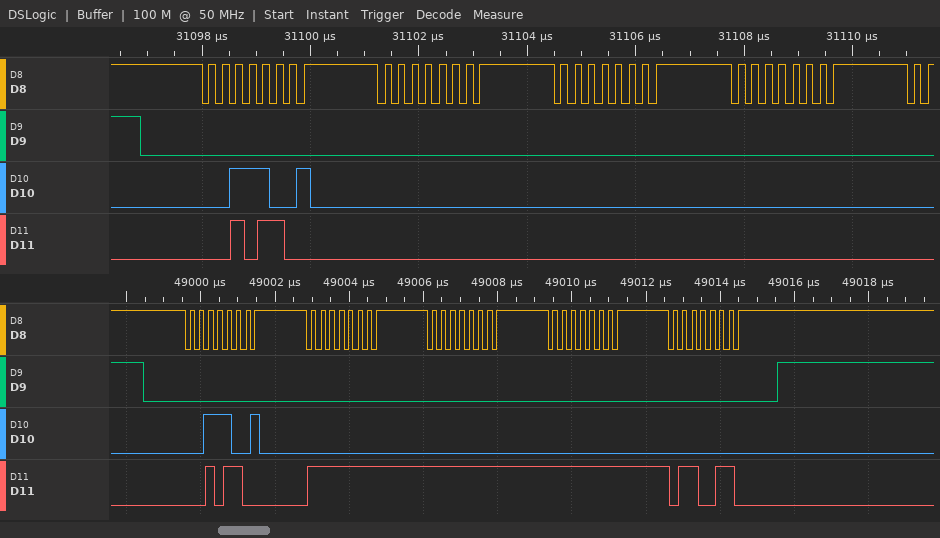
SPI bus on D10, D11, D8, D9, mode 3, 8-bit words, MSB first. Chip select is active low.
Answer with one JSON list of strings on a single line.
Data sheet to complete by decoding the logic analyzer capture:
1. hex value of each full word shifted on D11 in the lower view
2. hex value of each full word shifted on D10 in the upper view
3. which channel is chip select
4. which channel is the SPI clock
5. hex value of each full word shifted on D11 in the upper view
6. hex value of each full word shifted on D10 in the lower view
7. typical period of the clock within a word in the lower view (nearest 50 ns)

["2C, FF, FF, FF, 66", "39, 00, 00, 00", "D9", "D8", "2C, 00, 00, 00", "39, 00, 00, 00, 00", "250 ns"]
